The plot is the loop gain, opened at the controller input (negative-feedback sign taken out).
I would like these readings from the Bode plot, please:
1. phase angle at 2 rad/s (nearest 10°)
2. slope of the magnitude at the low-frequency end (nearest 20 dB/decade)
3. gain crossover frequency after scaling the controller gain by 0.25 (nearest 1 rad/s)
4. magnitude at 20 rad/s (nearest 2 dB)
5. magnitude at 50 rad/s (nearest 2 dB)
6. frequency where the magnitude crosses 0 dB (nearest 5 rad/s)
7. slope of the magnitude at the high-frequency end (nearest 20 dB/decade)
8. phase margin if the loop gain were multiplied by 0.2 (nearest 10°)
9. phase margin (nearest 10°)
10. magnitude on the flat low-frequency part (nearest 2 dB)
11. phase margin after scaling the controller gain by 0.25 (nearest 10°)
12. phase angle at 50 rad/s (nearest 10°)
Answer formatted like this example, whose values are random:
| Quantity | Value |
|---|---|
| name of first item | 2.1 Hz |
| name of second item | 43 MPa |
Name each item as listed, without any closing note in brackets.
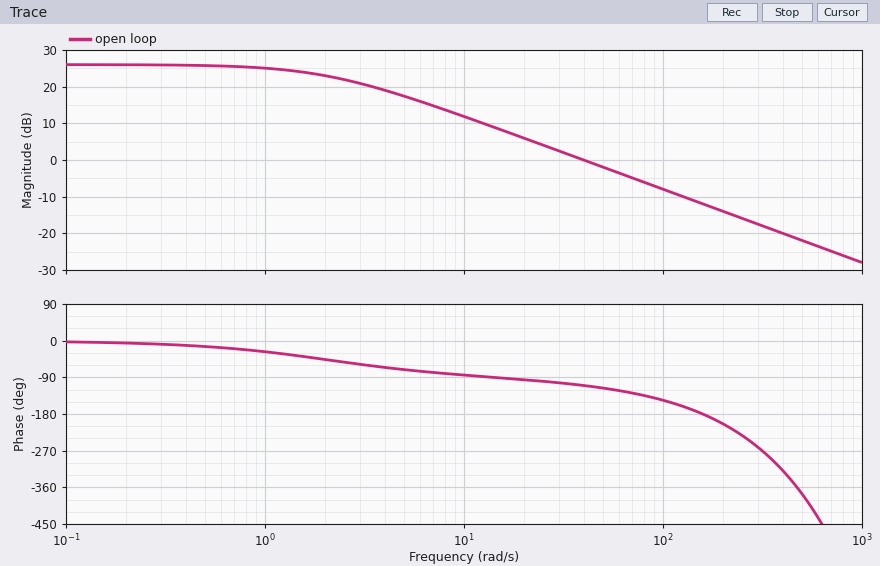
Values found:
| Quantity | Value |
|---|---|
| phase angle at 2 rad/s | -50° |
| slope of the magnitude at the low-frequency end | 0 dB/decade |
| gain crossover frequency after scaling the controller gain by 0.25 | 10 rad/s |
| magnitude at 20 rad/s | 6 dB |
| magnitude at 50 rad/s | -2 dB |
| frequency where the magnitude crosses 0 dB | 40 rad/s |
| slope of the magnitude at the high-frequency end | -20 dB/decade |
| phase margin if the loop gain were multiplied by 0.2 | 100° |
| phase margin | 70° |
| magnitude on the flat low-frequency part | 26 dB |
| phase margin after scaling the controller gain by 0.25 | 100° |
| phase angle at 50 rad/s | -120° |
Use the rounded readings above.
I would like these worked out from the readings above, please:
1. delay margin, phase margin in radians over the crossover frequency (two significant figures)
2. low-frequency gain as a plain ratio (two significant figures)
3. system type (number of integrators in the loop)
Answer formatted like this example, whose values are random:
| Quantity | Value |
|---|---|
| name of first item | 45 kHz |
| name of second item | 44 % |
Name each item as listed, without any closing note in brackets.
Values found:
| Quantity | Value |
|---|---|
| delay margin, phase margin in radians over the crossover frequency | 0.031 s |
| low-frequency gain as a plain ratio | 20 |
| system type | 0 |
